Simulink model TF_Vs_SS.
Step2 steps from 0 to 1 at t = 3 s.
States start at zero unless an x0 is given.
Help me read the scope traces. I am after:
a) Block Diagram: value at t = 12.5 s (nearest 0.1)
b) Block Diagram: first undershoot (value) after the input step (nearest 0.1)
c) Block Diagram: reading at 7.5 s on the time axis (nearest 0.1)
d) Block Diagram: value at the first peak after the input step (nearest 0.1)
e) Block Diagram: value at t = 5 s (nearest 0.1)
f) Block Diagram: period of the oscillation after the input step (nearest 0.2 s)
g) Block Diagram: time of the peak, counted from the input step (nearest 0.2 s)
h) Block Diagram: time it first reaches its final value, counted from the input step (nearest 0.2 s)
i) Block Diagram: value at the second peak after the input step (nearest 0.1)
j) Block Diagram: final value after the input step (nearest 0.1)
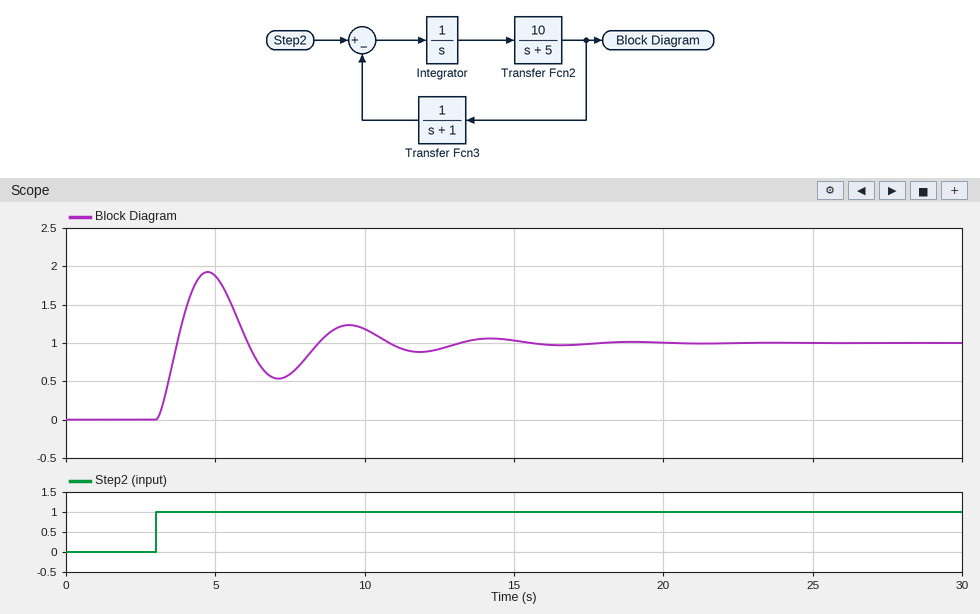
0.9
0.5
0.6
1.9
1.9
4.8 s
1.8 s
0.8 s
1.2
1.0
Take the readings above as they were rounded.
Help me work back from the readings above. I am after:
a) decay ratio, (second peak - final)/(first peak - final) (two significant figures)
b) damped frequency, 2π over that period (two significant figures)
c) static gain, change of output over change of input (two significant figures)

0.22
1.3 rad/s
1.0
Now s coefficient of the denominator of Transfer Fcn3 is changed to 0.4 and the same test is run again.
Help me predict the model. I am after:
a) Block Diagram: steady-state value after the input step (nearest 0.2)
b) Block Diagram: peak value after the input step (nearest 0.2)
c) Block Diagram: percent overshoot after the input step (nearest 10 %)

1.0
1.4
40 %
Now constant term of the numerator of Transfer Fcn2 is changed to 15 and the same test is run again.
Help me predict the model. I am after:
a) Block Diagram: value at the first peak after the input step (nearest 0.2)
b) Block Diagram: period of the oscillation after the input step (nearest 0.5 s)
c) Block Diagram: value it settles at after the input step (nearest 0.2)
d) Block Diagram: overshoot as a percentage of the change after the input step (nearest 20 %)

2.4
4.0 s
1.0
140 %
